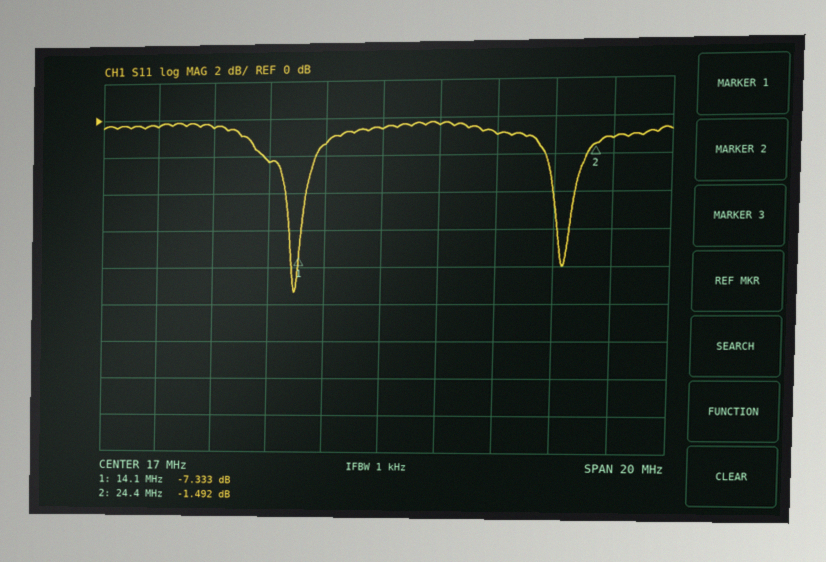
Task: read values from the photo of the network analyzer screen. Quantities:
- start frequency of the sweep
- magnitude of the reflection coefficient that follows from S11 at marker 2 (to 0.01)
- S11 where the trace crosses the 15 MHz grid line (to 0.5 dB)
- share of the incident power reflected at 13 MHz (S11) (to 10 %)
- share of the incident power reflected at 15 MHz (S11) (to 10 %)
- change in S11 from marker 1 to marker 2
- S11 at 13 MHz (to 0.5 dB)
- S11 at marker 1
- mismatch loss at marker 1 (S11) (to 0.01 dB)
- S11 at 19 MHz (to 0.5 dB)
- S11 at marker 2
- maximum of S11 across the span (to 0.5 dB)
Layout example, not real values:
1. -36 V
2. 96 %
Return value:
1. 7 MHz
2. 0.84
3. -1.5 dB
4. 60 %
5. 70 %
6. 5.841 dB
7. -2.5 dB
8. -7.333 dB
9. 0.89 dB
10. -0.5 dB
11. -1.492 dB
12. 0.0 dB
